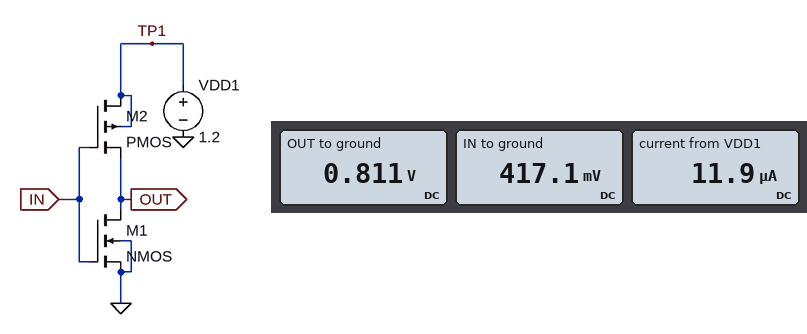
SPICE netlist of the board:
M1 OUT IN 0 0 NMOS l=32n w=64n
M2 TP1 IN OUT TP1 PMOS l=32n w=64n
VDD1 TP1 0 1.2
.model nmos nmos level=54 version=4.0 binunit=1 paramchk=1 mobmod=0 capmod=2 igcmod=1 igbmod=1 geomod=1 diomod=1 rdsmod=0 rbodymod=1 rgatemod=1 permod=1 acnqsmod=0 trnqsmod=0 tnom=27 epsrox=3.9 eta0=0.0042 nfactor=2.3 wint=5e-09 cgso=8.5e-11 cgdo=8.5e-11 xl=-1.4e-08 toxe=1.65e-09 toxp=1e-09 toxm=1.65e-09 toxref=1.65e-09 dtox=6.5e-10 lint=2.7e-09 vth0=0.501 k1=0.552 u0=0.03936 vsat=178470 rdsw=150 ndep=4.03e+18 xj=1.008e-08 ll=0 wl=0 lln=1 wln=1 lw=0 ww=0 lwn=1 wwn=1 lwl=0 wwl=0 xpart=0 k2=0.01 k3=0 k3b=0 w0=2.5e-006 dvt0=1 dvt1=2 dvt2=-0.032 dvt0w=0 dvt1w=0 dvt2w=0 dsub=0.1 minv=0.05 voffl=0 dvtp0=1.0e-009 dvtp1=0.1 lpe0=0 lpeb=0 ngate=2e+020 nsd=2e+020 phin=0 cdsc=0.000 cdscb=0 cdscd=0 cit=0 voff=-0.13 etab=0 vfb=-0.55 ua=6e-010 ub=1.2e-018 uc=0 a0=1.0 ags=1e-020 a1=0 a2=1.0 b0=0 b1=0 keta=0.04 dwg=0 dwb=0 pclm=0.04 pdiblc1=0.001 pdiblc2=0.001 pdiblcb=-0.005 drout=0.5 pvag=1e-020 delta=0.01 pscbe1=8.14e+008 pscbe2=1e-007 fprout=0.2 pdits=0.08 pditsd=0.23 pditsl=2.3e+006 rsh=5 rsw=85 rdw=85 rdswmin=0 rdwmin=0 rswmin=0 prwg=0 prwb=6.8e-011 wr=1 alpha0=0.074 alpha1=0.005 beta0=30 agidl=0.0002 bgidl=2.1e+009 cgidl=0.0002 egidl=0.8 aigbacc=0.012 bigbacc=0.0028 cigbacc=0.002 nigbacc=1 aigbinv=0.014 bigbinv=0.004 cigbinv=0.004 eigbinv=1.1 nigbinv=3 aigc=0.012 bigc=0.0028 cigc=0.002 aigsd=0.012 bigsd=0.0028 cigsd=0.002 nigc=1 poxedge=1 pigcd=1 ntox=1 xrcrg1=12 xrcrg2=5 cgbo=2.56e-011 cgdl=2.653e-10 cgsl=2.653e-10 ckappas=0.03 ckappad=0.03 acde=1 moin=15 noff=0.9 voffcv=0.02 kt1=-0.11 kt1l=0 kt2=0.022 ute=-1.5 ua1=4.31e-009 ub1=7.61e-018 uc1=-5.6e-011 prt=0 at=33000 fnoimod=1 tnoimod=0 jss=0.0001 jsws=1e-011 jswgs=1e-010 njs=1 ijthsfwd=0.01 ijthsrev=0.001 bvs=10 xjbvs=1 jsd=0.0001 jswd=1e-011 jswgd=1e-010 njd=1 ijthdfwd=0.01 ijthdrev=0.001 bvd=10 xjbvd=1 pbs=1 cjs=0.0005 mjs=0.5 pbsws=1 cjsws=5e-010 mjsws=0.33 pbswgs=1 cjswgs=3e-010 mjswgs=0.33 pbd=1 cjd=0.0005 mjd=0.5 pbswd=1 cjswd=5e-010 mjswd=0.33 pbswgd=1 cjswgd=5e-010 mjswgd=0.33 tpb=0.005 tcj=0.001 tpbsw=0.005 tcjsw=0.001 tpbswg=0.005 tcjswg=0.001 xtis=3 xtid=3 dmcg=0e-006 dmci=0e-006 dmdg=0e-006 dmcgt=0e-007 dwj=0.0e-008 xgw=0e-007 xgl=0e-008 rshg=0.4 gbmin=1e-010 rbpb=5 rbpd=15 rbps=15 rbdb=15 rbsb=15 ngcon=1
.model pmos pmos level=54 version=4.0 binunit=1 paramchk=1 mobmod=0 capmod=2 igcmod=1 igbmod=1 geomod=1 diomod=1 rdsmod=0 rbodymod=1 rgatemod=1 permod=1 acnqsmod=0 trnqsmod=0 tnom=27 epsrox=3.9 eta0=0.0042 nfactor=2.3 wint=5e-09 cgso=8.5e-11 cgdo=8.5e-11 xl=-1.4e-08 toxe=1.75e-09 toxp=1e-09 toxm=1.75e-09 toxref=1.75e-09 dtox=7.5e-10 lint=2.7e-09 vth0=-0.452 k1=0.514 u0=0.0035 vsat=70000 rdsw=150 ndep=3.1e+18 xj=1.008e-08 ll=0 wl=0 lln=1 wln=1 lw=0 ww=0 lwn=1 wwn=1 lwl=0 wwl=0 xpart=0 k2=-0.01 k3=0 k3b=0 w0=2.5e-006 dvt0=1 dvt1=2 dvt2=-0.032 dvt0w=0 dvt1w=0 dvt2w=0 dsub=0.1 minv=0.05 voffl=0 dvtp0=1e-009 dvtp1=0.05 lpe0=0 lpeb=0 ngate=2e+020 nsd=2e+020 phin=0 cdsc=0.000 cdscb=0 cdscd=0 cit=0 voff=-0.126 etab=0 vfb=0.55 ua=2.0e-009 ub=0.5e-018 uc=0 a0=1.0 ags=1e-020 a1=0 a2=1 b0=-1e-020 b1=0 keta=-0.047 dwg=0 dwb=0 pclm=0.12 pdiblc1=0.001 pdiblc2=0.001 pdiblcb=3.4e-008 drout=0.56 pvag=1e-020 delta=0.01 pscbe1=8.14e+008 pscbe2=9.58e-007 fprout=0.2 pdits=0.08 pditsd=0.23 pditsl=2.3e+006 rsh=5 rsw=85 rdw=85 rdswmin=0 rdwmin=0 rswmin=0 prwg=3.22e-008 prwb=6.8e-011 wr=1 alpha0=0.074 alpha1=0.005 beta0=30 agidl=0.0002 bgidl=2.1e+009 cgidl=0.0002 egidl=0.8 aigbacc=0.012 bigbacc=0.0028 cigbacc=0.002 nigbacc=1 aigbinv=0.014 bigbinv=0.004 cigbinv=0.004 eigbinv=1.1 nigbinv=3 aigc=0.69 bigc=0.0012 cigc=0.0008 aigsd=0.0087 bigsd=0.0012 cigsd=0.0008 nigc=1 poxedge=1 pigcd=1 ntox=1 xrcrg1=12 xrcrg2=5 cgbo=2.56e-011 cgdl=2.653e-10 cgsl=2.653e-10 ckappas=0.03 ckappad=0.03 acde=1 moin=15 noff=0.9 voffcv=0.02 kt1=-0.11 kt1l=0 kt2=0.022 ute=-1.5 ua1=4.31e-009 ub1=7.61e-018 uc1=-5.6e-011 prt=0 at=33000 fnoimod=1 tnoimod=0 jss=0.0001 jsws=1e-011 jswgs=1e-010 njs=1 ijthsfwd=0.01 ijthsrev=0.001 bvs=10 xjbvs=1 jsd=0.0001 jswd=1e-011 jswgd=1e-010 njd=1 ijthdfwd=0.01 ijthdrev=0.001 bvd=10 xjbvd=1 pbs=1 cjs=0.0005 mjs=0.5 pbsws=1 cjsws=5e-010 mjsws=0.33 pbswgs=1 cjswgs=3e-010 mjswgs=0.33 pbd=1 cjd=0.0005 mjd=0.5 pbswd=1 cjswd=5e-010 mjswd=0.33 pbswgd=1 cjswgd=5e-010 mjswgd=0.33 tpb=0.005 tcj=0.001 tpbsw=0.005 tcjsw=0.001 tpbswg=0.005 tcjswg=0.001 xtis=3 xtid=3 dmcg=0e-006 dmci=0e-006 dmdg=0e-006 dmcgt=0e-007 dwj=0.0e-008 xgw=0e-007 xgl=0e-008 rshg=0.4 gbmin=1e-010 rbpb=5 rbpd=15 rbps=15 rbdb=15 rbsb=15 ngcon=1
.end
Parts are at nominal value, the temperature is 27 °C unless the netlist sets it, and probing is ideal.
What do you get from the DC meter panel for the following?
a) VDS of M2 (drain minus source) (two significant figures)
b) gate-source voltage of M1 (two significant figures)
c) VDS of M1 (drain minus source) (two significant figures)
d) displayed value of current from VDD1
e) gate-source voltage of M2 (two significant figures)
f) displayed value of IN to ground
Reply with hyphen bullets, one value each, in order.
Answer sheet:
- 390 mV
- 420 mV
- 810 mV
- 11.9 µA
- -390 mV
- 417.1 mV
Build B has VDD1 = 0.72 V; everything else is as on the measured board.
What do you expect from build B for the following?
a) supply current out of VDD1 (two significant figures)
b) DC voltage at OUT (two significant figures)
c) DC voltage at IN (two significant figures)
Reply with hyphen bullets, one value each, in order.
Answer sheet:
- 630 nA
- 540 mV
- 270 mV
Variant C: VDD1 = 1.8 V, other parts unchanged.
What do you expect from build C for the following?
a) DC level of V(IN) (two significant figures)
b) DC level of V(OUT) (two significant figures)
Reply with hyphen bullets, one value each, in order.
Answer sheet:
- 570 mV
- 1.1 V
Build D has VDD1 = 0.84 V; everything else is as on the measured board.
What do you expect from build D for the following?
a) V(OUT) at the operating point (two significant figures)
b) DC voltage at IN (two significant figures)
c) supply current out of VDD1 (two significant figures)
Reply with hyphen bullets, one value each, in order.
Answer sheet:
- 620 mV
- 320 mV
- 1.9 µA
